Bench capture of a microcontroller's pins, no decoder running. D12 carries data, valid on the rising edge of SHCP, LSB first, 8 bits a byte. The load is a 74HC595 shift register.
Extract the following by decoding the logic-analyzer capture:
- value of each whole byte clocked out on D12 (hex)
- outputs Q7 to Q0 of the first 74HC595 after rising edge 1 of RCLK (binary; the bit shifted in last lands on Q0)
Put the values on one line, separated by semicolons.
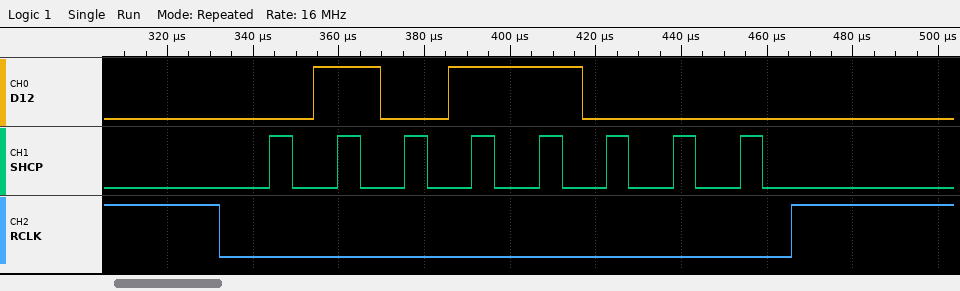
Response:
1A; 01011000
